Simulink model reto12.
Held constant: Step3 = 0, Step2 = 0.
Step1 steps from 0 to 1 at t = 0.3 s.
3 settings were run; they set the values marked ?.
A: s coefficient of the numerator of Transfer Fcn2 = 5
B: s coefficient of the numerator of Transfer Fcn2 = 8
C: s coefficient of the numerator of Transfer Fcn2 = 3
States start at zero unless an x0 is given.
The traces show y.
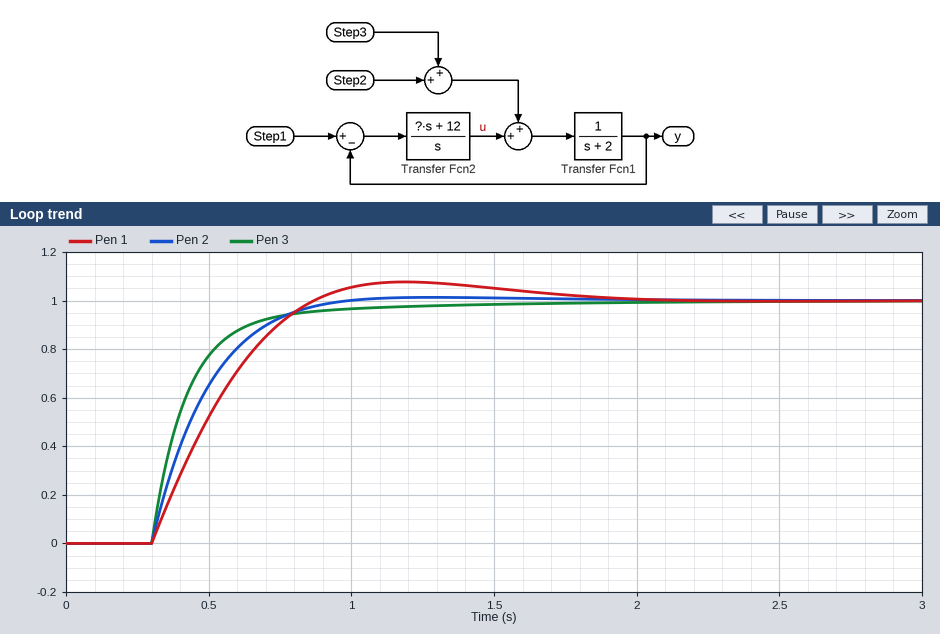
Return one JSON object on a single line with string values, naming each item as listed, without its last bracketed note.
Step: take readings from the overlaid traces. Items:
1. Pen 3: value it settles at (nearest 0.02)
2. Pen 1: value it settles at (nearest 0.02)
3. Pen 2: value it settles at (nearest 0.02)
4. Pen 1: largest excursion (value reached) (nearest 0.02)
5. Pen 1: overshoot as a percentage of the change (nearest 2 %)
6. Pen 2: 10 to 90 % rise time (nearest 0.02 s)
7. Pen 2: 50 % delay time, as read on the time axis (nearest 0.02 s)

{"Pen 3: value it settles at": "1.00", "Pen 1: value it settles at": "1.00", "Pen 2: value it settles at": "1.00", "Pen 1: largest excursion (value reached)": "1.08", "Pen 1: overshoot as a percentage of the change": "8 %", "Pen 2: 10 to 90 % rise time": "0.38 s", "Pen 2: 50 % delay time, as read on the time axis": "0.44 s"}
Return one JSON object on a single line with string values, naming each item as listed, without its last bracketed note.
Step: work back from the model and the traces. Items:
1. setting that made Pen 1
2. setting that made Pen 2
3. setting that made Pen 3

{"setting that made Pen 1": "C", "setting that made Pen 2": "A", "setting that made Pen 3": "B"}
